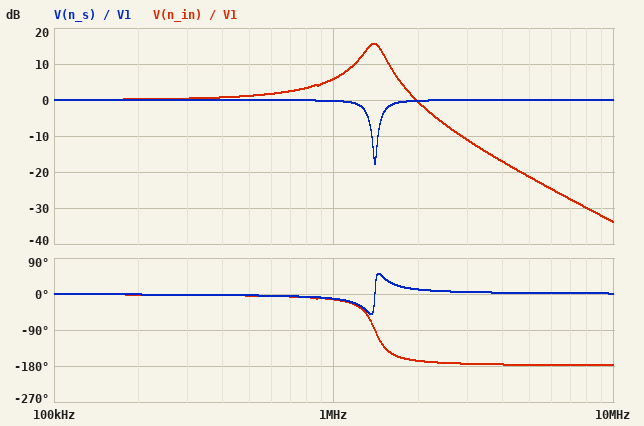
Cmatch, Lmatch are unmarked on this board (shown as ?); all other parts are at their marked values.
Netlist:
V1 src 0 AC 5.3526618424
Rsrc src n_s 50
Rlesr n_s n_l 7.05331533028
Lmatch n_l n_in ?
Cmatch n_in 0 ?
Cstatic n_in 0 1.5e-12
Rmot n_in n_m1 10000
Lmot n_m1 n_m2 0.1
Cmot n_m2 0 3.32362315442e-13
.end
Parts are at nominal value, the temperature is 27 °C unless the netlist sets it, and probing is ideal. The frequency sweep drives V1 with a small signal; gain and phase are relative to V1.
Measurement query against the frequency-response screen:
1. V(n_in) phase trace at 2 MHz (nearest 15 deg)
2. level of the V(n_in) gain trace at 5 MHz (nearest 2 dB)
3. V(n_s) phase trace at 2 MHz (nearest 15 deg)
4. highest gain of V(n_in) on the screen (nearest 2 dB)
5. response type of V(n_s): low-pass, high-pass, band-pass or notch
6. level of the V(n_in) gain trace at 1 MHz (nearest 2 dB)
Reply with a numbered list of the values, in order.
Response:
1. -165 deg
2. -22 dB
3. 15 deg
4. 16 dB
5. notch
6. 6 dB
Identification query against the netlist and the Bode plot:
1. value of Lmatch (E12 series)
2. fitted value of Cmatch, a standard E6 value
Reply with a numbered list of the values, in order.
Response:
1. 39 µH
2. 330 pF
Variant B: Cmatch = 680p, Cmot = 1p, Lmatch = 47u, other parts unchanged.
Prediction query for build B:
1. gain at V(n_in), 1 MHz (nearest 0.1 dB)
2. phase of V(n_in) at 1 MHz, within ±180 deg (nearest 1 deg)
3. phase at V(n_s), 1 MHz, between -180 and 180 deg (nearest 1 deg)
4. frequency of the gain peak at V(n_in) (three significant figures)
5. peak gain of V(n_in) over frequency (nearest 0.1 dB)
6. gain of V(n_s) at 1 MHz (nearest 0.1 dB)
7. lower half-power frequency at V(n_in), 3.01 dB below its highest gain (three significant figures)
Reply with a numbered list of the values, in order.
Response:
1. 8.9 dB
2. -137 deg
3. 36 deg
4. 879 kHz
5. 13.3 dB
6. -2.6 dB
7. 776 kHz
